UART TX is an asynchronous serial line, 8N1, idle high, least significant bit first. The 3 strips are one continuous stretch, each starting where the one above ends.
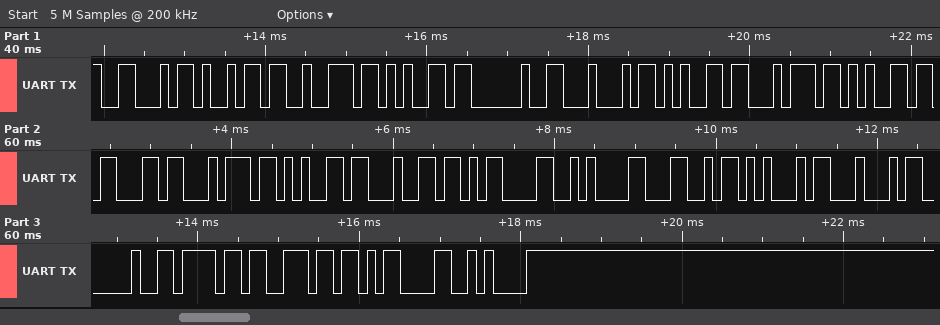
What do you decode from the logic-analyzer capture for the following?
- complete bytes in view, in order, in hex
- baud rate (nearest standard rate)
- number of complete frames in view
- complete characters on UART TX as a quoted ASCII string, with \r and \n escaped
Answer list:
46 69 72 65 20 44 65 74 65 63 74 65 64 0D 0A 4C 45 44 20 6F 6E 0D 0A
9600 baud
23
"Fire Detected\r\nLED on\r\n"
